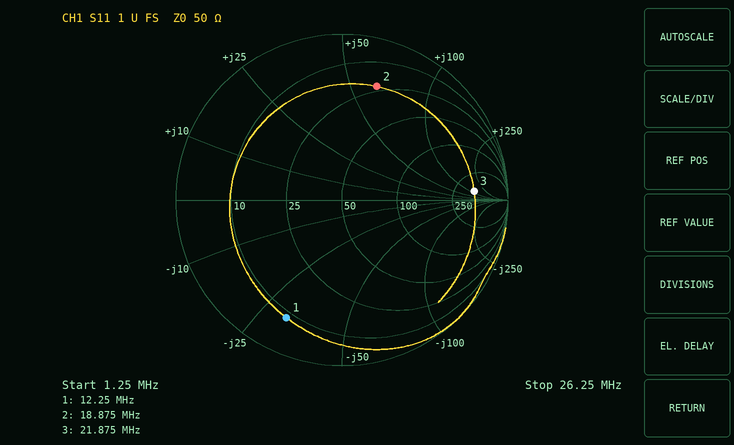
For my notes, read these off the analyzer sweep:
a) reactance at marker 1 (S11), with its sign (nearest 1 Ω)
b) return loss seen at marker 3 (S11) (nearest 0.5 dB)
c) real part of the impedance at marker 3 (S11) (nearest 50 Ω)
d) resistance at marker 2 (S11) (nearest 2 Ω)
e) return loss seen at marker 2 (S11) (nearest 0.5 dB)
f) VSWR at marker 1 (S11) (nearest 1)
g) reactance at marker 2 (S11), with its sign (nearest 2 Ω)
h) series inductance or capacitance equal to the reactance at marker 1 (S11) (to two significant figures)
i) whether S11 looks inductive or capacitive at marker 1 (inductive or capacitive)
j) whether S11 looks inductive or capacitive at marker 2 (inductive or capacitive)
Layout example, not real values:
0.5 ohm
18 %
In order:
-31 Ω
2.0 dB
400 Ω
22 Ω
3.0 dB
8
+62 Ω
420 pF
capacitive
inductive
